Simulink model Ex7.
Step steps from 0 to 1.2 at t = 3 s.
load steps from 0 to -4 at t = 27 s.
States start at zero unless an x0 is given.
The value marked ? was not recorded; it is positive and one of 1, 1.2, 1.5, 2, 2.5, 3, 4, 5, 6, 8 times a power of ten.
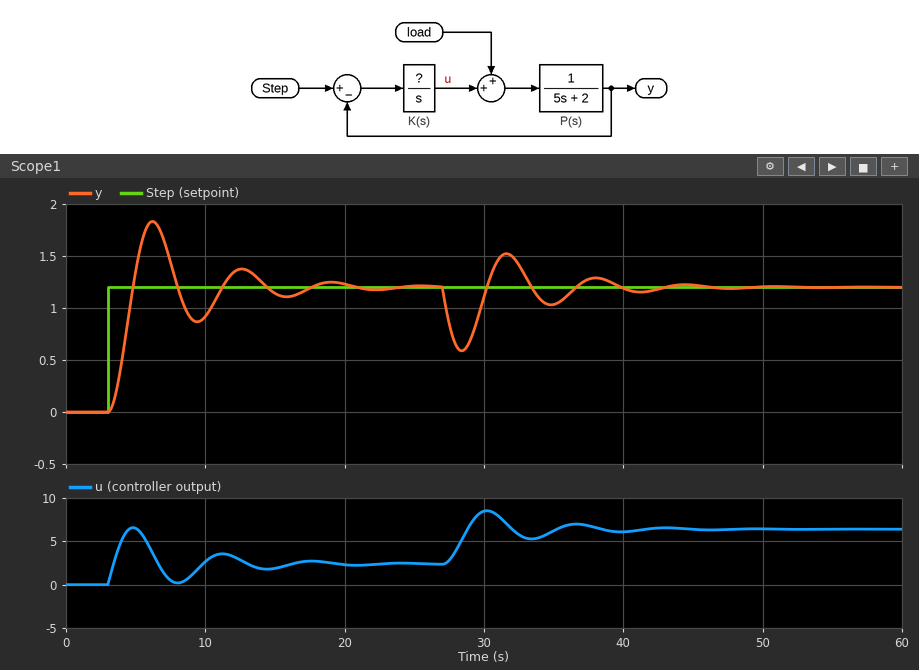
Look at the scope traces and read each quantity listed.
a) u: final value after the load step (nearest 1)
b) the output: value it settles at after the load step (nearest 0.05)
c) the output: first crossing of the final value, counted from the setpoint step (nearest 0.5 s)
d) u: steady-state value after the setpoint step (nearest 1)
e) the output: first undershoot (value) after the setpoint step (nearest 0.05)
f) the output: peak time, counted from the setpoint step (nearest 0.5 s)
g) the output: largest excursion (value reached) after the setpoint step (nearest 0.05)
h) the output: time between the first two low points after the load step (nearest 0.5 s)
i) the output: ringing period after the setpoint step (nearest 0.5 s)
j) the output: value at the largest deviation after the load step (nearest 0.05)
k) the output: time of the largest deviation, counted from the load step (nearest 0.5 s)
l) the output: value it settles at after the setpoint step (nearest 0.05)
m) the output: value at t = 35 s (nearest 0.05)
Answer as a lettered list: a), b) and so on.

a) 6
b) 1.20
c) 2.0 s
d) 2
e) 0.85
f) 3.0 s
g) 1.85
h) 6.5 s
i) 6.5 s
j) 0.60
k) 1.5 s
l) 1.20
m) 1.05
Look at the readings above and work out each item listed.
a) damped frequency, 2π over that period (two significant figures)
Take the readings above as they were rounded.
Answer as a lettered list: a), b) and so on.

a) 0.97 rad/s
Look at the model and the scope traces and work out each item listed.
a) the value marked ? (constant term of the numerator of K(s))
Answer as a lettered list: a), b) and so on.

a) 5
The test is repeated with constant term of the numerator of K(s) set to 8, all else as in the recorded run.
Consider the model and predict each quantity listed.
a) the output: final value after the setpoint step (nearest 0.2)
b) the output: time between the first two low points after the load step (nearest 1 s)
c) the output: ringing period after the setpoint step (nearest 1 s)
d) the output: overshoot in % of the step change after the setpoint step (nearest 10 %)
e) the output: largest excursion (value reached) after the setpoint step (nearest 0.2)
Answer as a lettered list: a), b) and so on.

a) 1.2
b) 5 s
c) 5 s
d) 60 %
e) 2.0
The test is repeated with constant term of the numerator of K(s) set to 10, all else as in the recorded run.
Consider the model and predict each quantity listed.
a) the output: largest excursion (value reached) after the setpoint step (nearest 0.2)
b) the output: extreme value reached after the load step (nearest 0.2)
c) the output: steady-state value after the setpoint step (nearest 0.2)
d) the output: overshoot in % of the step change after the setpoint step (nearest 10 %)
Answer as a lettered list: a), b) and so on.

a) 2.0
b) 0.8
c) 1.2
d) 60 %
